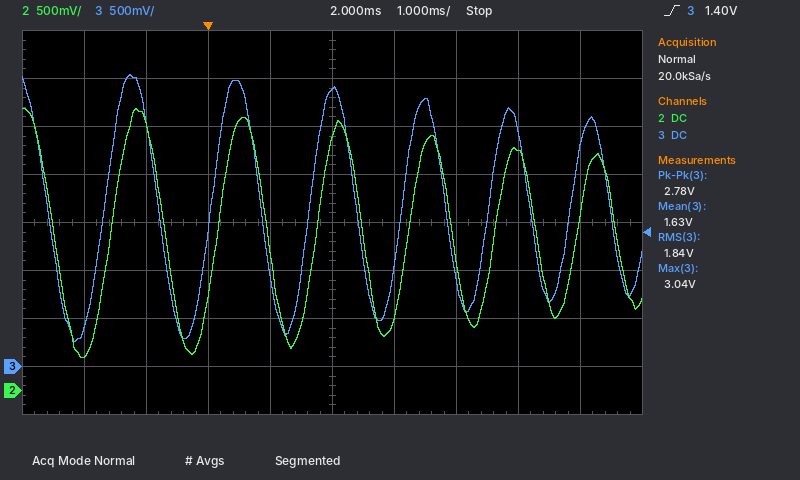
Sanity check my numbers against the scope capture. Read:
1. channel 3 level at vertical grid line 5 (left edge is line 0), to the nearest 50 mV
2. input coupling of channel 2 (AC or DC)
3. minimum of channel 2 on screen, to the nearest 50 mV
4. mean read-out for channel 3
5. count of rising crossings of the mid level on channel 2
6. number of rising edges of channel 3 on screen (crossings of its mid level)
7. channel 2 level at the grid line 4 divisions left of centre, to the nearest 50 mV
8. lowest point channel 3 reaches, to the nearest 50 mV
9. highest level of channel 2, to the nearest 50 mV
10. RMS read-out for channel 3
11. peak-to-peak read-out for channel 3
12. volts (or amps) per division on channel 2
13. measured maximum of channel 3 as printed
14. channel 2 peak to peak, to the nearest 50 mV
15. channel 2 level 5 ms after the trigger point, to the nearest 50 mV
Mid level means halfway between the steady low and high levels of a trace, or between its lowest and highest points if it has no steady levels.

2.90 V
DC
350 mV
1.63 V
6
6
350 mV
250 mV
2.95 V
1.84 V
2.78 V
500 mV
3.04 V
2.60 V
2.50 V
